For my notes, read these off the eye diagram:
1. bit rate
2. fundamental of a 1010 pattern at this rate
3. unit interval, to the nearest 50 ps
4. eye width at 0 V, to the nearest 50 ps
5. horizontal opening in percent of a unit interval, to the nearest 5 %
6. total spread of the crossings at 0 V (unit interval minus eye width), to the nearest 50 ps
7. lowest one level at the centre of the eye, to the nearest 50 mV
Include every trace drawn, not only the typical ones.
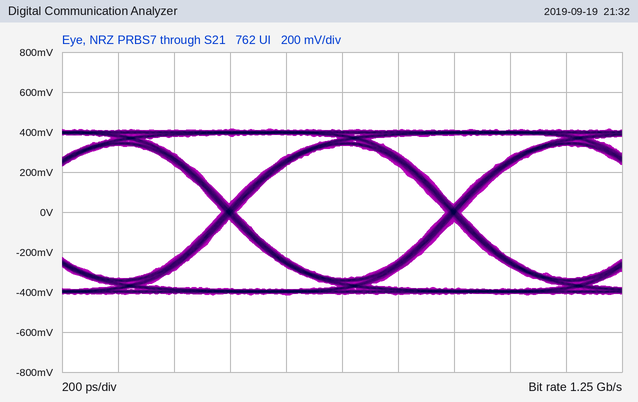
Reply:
1.25 Gb/s
625 MHz
800 ps
750 ps
95 %
50 ps
350 mV
